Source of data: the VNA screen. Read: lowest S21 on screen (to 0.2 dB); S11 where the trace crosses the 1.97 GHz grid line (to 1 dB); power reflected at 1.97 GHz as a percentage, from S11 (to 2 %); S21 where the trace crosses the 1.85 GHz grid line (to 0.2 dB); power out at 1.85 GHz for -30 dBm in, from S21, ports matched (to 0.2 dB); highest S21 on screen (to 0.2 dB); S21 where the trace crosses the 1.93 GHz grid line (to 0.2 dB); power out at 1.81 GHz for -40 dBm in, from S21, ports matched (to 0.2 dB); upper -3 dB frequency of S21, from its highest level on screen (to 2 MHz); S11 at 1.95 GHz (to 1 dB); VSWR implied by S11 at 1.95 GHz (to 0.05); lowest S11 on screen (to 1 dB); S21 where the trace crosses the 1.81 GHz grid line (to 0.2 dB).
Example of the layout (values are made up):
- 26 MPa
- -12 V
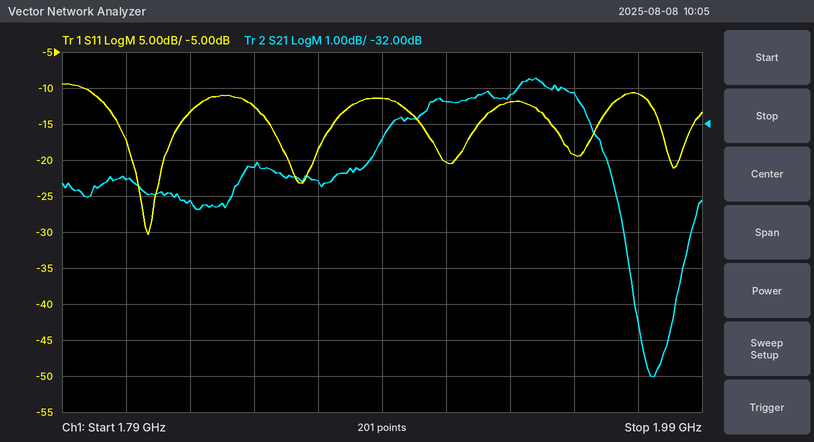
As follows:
- -39.0 dB
- -11 dB
- 8 %
- -33.2 dB
- -63.2 dBm
- -30.8 dB
- -31.2 dB
- -73.6 dBm
- 1.962 GHz
- -19 dB
- 1.25
- -30 dB
- -33.6 dB
